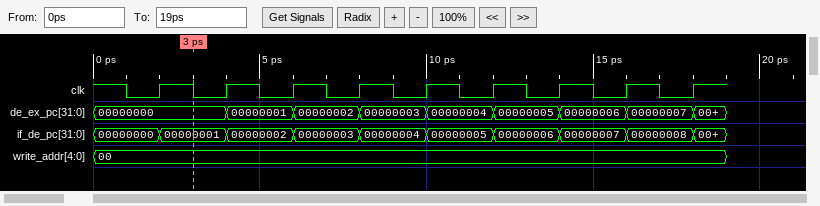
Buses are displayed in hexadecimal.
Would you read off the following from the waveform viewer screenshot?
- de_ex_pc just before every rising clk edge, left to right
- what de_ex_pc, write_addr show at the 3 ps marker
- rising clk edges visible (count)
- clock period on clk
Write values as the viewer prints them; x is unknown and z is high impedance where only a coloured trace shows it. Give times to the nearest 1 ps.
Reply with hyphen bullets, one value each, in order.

- 00000000, 00000000, 00000001, 00000002, 00000003, 00000004, 00000005, 00000006, 00000007
- de_ex_pc=00000000, write_addr=00
- 9
- 2 ps
